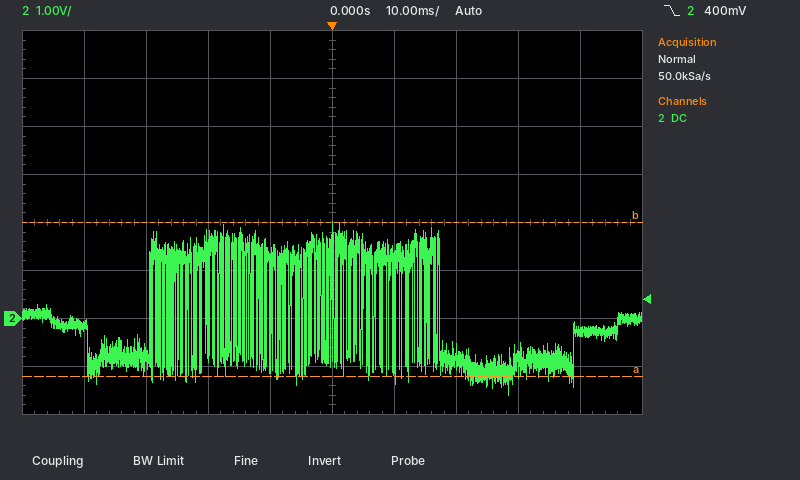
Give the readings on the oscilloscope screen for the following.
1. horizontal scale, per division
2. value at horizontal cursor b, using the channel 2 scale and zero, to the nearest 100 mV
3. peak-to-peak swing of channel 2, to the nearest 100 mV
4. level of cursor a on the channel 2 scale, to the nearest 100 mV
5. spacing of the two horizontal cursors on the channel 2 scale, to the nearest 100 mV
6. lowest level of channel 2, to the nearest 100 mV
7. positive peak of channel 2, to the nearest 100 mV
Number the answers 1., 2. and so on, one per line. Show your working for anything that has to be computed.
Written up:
1. 10 ms
2. 2.0 V
3. 2.0 V − (-1.6 V) = 3.6 V
4. -1.2 V
5. 3.2 V
6. -1.6 V
7. 2.0 V
